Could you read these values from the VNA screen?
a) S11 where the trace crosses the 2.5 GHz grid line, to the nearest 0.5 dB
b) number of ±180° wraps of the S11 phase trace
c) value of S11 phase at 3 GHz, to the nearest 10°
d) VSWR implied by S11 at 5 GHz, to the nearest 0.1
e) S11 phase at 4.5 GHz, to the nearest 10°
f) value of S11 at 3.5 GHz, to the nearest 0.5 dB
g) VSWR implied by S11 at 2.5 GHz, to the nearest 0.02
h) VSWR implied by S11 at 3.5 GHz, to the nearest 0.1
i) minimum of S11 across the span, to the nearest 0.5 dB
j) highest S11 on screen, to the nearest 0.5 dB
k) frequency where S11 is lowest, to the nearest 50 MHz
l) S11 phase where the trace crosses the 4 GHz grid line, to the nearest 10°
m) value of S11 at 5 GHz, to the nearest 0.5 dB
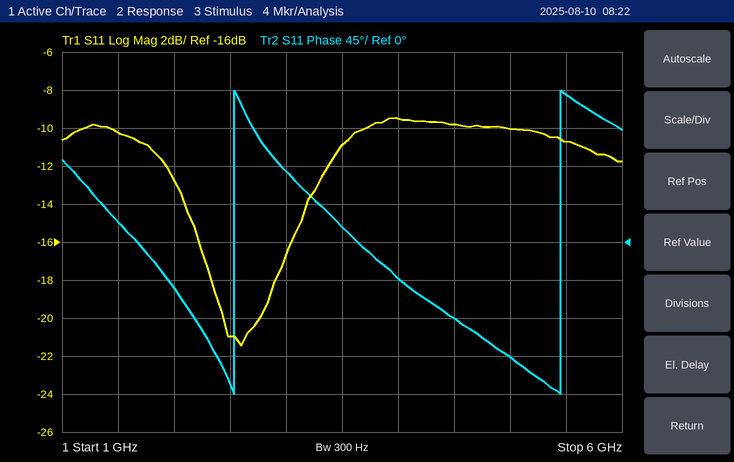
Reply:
-21.0 dB
2
80°
1.9
-90°
-11.0 dB
1.20
1.8
-21.5 dB
-9.5 dB
2.60 GHz
-40°
-10.0 dB
